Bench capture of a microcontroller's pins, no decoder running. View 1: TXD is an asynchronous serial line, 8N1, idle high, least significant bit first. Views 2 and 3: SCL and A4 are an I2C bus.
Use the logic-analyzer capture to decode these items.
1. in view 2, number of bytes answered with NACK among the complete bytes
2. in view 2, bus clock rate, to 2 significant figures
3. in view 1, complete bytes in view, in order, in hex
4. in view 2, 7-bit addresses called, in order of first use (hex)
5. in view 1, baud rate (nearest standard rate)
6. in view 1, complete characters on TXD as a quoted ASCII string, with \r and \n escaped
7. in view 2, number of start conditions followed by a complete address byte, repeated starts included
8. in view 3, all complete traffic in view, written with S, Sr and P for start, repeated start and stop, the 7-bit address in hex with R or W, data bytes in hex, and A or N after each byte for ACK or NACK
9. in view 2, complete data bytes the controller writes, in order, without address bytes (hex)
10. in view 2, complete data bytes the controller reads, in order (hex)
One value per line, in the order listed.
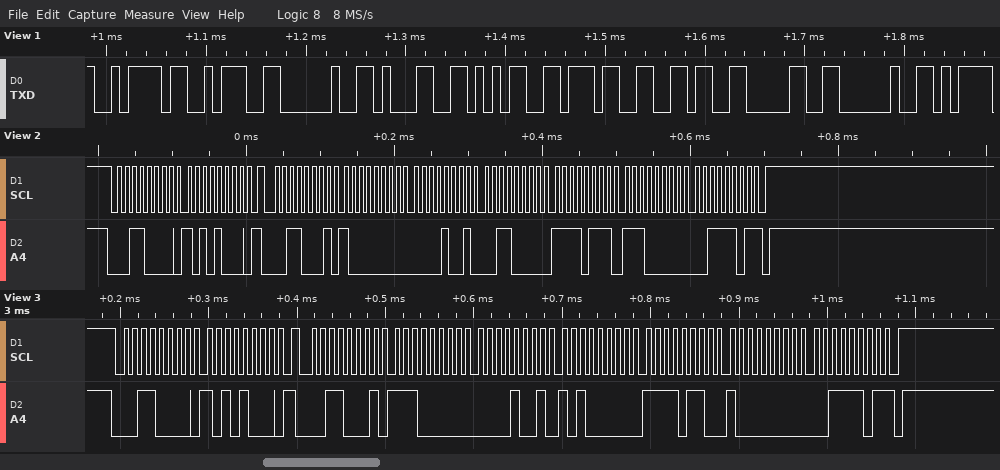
1
100 kHz
0x7A 0x3A 0x20 0x31 0x35 0x37 0x36 0x30 0x20
0x18
115200 baud
"z: 15760 "
2
S 18W A A8 A Sr 18R A E0 A 09 A A0 A F6 A 80 A 3D N P
A8
80 09 30 F7 E0 3D
